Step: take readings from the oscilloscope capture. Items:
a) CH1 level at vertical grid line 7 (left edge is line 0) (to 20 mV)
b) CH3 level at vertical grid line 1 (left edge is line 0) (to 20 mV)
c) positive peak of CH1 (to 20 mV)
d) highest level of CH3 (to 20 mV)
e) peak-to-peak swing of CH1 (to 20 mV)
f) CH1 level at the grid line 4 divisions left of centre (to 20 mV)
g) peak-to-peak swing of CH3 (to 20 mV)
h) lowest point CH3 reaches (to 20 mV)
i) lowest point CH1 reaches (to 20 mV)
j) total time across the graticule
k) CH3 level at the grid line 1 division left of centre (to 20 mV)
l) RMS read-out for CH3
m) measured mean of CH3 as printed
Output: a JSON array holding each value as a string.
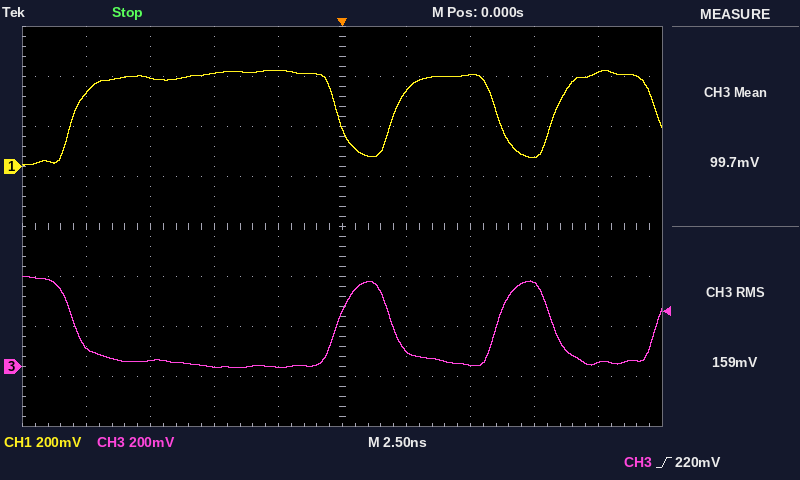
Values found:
["360 mV", "80 mV", "380 mV", "360 mV", "380 mV", "300 mV", "360 mV", "0 mV", "0 mV", "25 ns", "0 mV", "159 mV", "99.7 mV"]
